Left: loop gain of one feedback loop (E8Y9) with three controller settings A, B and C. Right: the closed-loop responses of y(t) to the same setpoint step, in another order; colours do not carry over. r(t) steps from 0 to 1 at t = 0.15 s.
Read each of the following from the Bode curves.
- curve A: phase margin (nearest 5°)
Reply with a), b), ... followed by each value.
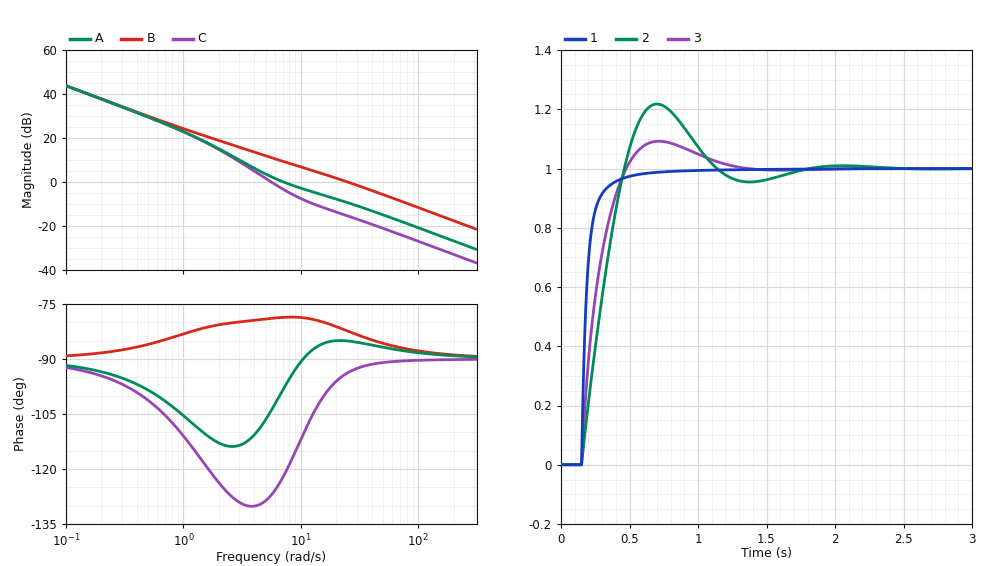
a) 80°
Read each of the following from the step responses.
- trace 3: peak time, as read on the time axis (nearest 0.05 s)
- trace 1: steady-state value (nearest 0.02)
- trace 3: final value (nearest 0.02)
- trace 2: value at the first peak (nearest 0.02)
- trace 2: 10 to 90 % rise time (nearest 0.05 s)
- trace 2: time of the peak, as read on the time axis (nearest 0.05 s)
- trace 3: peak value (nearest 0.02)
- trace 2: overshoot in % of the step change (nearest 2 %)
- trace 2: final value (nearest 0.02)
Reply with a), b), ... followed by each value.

a) 0.70 s
b) 1.00
c) 1.00
d) 1.22
e) 0.25 s
f) 0.70 s
g) 1.10
h) 22 %
i) 1.00
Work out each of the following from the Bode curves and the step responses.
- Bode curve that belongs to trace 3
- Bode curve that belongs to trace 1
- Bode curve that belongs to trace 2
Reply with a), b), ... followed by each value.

a) A
b) B
c) C
